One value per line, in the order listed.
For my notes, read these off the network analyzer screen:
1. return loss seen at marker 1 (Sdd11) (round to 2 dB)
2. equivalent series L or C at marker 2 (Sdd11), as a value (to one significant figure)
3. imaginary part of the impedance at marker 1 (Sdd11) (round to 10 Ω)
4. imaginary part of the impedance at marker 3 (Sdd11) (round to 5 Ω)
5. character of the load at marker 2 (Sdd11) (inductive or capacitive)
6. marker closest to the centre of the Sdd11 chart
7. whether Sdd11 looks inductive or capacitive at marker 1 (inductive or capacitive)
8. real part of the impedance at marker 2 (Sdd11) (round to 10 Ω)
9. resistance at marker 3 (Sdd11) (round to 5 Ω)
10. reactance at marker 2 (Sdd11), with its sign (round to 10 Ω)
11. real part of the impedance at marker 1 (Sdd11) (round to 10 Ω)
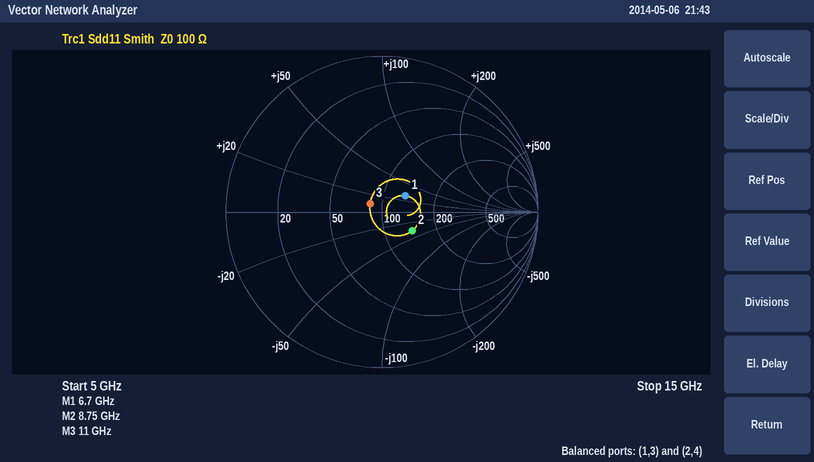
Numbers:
14 dB
500 fF
+30 Ω
+10 Ω
capacitive
marker 3
inductive
140 Ω
85 Ω
-40 Ω
130 Ω
